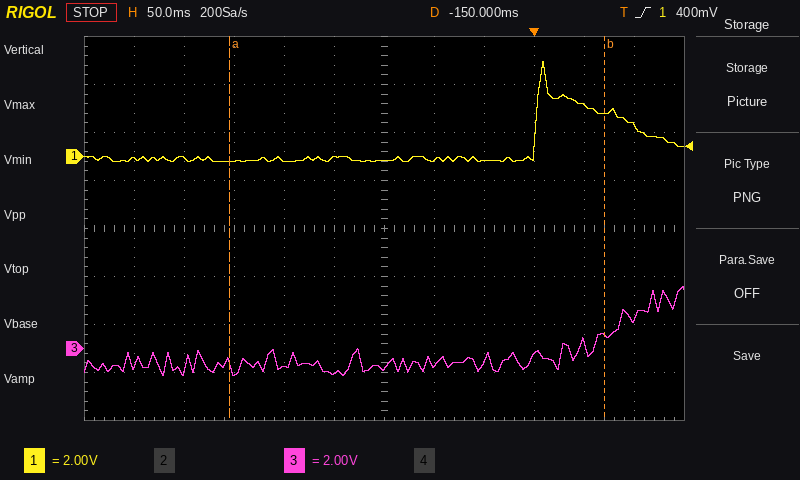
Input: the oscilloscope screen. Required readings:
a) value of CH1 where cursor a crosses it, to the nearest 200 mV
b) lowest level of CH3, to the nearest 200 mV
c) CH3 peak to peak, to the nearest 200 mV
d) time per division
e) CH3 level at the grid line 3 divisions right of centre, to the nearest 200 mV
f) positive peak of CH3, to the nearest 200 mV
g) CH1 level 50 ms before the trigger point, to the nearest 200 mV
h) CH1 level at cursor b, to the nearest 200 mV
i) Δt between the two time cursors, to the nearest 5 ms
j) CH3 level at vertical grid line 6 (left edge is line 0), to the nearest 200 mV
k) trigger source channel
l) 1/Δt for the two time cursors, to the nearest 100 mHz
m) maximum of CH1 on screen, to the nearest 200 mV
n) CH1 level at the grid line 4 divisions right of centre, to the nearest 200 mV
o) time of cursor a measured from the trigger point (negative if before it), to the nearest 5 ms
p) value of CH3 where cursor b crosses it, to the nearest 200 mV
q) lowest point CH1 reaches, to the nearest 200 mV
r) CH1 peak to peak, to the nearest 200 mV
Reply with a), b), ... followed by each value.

a) -200 mV
b) -1.2 V
c) 3.8 V
d) 50 ms
e) -200 mV
f) 2.6 V
g) -200 mV
h) 1.8 V
i) 375 ms
j) -800 mV
k) CH1
l) 2.7 Hz
m) 4.0 V
n) 2.2 V
o) -305 ms
p) 600 mV
q) -200 mV
r) 4.2 V
